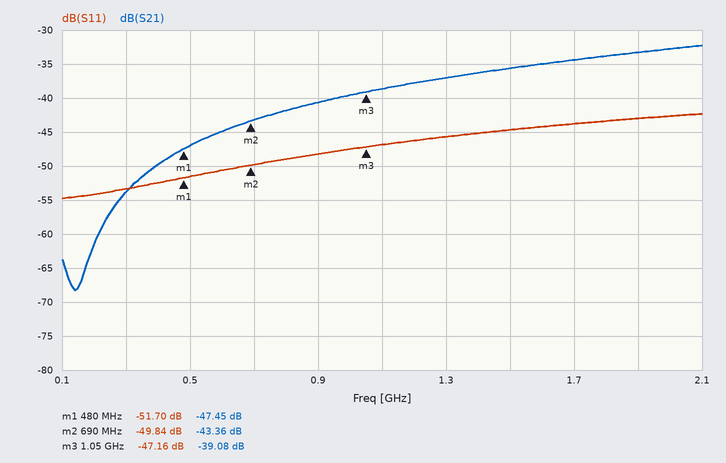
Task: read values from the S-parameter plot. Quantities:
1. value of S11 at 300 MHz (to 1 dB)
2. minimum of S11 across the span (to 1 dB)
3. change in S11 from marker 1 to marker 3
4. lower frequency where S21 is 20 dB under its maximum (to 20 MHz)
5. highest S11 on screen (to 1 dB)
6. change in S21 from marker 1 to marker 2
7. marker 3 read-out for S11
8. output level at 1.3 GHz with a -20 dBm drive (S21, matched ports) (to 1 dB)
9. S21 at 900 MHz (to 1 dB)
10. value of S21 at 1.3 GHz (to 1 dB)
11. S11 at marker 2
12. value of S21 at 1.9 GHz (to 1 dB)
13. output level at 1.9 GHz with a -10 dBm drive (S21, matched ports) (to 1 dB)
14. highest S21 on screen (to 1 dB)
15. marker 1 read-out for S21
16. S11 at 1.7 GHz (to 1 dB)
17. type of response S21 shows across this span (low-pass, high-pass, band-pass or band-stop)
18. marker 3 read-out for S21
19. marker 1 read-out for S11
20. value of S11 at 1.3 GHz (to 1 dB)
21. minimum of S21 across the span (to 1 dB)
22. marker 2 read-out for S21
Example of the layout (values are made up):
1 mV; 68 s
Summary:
-53 dB; -55 dB; 4.54 dB; 340 MHz; -42 dB; 4.09 dB; -47.16 dB; -57 dBm; -41 dB; -37 dB; -49.84 dB; -33 dB; -43 dBm; -32 dB; -47.45 dB; -44 dB; high-pass; -39.08 dB; -51.70 dB; -46 dB; -68 dB; -43.36 dB
